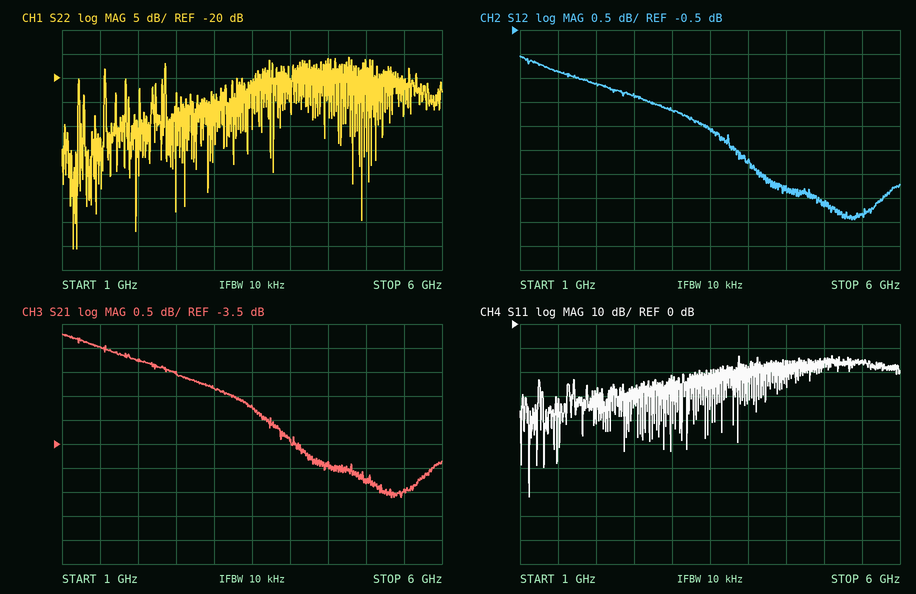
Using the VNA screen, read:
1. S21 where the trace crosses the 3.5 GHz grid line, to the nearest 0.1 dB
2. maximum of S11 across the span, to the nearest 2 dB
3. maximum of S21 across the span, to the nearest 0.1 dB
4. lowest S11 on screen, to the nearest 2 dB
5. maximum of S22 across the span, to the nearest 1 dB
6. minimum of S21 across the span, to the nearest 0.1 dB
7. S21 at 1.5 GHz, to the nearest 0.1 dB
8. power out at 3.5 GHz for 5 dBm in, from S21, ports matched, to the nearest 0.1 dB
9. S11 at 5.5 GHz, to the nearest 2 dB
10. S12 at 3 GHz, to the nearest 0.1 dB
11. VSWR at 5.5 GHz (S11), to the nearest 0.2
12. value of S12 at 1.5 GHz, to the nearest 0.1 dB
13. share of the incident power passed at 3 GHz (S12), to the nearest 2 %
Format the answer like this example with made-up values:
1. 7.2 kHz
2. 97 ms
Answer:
1. -2.7 dB
2. -14 dB
3. -1.2 dB
4. -72 dB
5. -16 dB
6. -4.6 dB
7. -1.5 dB
8. 2.3 dBm
9. -16 dB
10. -2.2 dB
11. 1.4
12. -1.4 dB
13. 60 %
